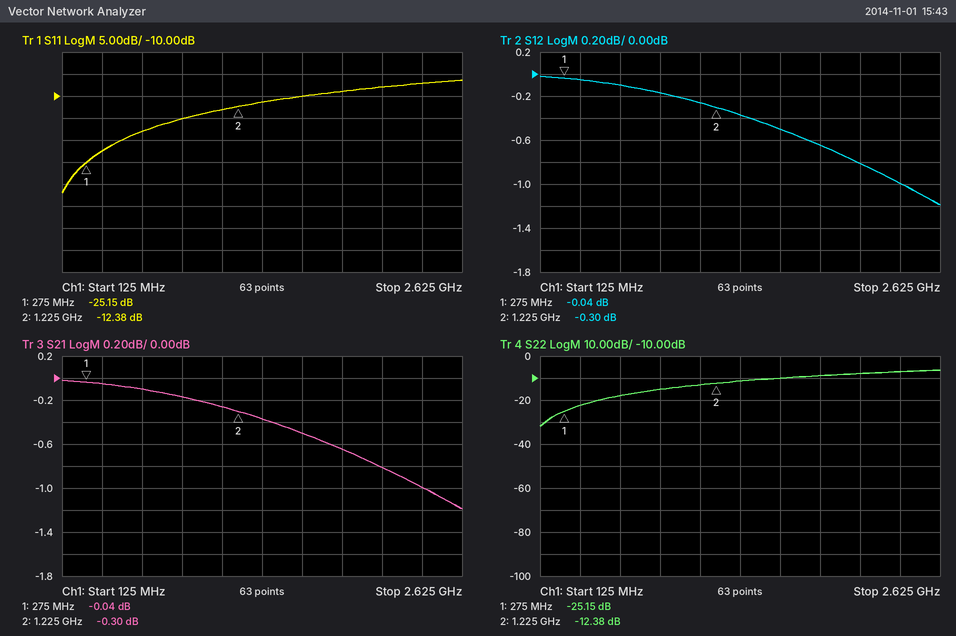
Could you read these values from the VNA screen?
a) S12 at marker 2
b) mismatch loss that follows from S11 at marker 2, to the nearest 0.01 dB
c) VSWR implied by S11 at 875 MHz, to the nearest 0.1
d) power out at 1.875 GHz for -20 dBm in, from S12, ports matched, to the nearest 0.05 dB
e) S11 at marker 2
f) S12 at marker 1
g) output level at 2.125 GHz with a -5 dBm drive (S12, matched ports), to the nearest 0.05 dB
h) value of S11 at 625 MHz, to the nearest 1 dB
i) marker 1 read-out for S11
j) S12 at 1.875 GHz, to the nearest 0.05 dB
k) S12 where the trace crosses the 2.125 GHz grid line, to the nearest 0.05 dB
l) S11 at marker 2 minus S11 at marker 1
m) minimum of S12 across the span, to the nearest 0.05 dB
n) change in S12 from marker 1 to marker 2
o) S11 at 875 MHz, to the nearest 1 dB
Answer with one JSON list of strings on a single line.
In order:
["-0.30 dB", "0.26 dB", "1.4", "-20.65 dBm", "-12.38 dB", "-0.04 dB", "-5.80 dBm", "-18 dB", "-25.15 dB", "-0.65 dB", "-0.80 dB", "12.77 dB", "-1.20 dB", "-0.26 dB", "-15 dB"]
